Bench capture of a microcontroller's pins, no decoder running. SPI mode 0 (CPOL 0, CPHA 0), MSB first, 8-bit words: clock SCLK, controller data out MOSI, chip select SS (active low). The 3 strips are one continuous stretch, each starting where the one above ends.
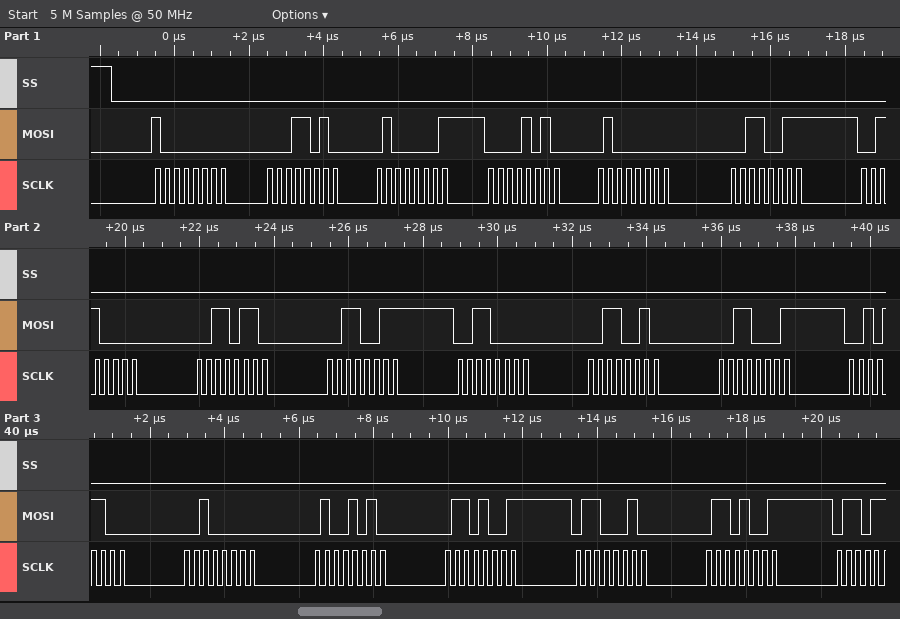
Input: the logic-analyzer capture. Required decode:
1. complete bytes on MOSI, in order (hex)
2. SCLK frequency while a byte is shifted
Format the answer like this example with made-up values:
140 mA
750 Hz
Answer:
80 1A 41 0A 40 33 30 36 33 30 32 31 2C 20 4A 69 62 69
4 MHz
